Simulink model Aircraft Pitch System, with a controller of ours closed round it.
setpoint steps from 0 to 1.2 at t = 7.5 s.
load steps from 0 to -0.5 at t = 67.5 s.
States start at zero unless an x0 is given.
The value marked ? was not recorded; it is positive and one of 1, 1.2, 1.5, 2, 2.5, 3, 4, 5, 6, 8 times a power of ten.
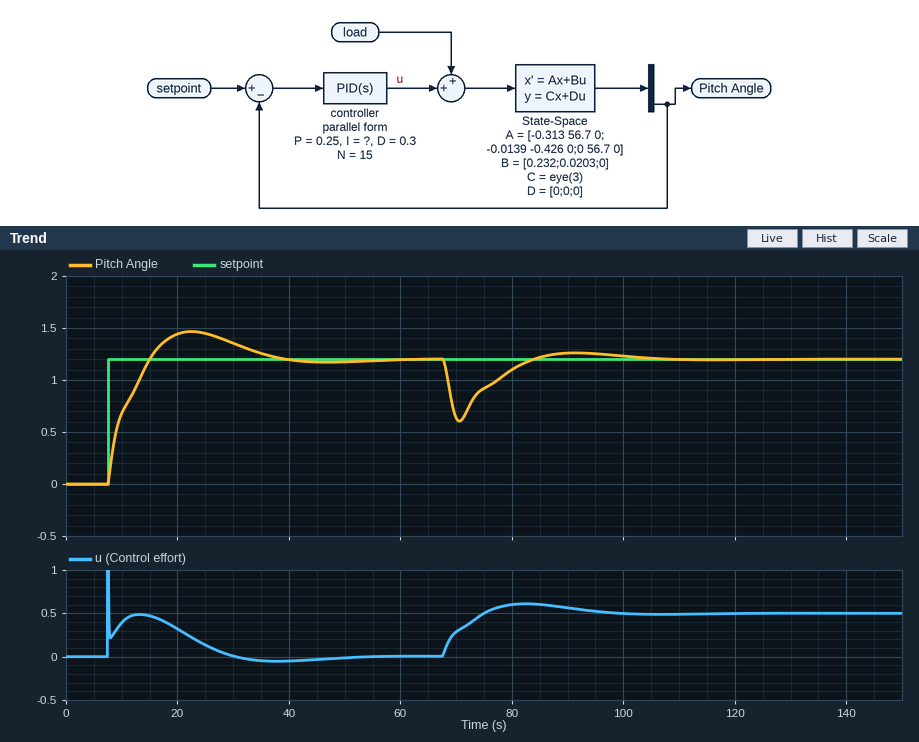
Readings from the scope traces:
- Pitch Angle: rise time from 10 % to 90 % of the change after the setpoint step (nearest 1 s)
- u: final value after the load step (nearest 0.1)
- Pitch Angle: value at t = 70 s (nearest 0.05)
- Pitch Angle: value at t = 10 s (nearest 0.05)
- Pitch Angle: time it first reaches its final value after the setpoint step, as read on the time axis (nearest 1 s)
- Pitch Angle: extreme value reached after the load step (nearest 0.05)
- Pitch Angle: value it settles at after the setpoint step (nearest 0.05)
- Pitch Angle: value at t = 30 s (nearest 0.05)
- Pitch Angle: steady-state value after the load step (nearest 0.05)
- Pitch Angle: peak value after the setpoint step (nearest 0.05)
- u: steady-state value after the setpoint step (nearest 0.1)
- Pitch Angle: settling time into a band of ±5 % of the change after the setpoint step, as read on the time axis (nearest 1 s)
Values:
6 s
0.5
0.65
0.70
15 s
0.60
1.20
1.35
1.20
1.45
0.0
35 s
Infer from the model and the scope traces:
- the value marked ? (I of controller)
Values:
0.15
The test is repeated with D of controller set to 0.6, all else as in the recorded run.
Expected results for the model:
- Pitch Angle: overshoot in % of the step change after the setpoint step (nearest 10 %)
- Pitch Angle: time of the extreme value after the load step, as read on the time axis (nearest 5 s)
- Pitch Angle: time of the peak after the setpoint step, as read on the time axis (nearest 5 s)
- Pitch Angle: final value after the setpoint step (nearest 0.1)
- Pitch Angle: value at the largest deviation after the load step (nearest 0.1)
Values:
20 %
70 s
25 s
1.2
0.7
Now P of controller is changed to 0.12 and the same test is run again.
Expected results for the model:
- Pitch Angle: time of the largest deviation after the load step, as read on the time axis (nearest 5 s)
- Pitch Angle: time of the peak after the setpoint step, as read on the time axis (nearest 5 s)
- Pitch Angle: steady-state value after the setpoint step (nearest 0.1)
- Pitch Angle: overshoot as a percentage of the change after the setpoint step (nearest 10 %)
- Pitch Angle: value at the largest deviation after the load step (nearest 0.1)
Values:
70 s
20 s
1.2
30 %
0.5
